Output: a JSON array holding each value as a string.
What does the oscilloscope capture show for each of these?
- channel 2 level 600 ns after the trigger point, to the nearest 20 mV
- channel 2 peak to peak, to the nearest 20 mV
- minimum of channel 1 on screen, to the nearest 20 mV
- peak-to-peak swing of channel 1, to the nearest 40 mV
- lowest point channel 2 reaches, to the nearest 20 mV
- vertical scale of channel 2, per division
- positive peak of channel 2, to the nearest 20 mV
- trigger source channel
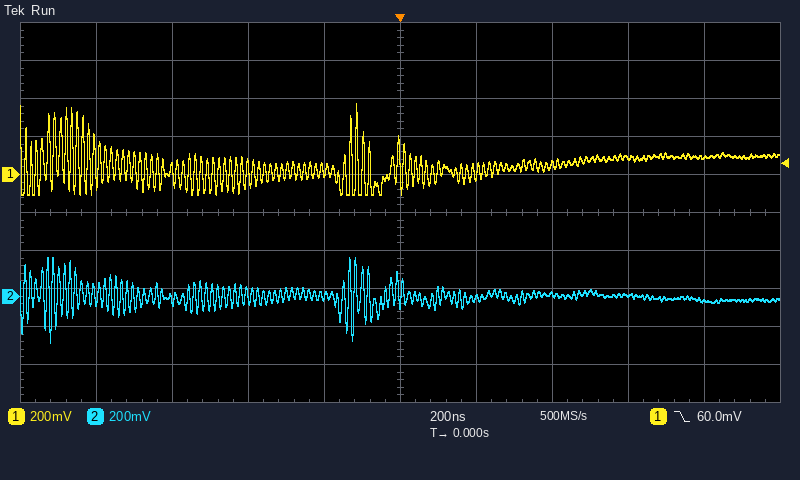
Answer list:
["0 mV", "440 mV", "-100 mV", "480 mV", "-240 mV", "200 mV", "200 mV", "channel 1"]
